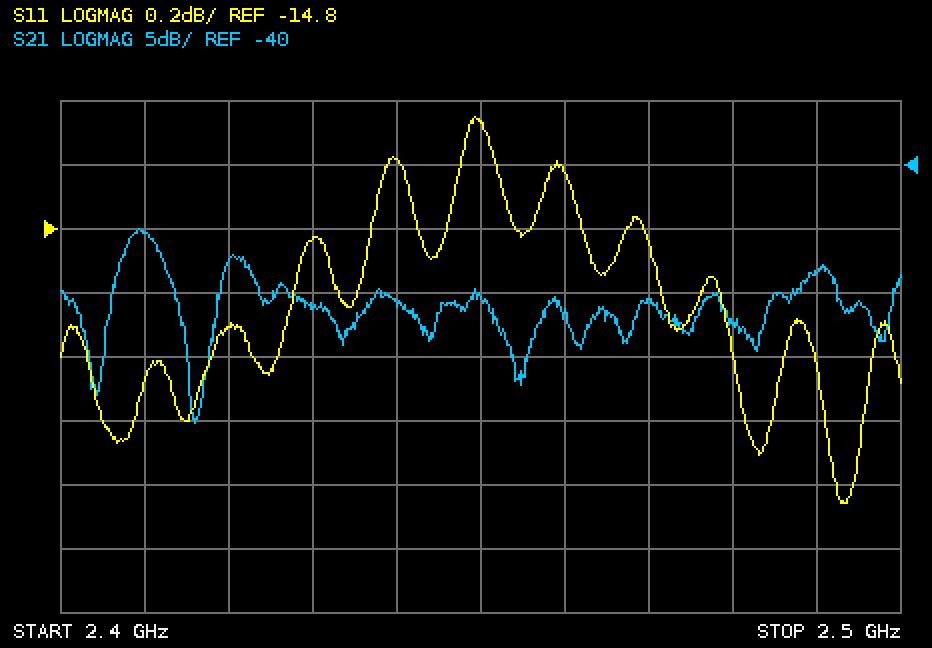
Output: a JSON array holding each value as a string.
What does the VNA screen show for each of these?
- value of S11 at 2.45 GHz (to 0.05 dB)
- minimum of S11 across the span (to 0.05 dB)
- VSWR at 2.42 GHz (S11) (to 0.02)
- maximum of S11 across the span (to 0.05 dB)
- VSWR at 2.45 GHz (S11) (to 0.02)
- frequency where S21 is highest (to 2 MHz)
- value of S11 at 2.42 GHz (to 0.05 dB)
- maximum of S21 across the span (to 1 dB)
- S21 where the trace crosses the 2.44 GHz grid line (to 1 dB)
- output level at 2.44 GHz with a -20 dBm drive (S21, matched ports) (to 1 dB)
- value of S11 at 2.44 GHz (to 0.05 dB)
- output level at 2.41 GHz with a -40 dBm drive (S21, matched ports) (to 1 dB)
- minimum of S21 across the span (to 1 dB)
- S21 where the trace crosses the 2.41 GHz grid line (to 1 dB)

["-14.45 dB", "-15.65 dB", "1.42", "-14.45 dB", "1.46", "2.410 GHz", "-15.10 dB", "-45 dB", "-51 dB", "-71 dBm", "-14.60 dB", "-85 dBm", "-60 dB", "-45 dB"]
